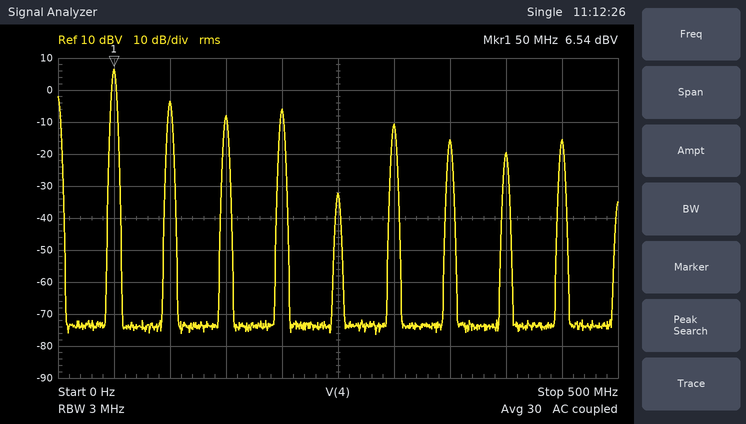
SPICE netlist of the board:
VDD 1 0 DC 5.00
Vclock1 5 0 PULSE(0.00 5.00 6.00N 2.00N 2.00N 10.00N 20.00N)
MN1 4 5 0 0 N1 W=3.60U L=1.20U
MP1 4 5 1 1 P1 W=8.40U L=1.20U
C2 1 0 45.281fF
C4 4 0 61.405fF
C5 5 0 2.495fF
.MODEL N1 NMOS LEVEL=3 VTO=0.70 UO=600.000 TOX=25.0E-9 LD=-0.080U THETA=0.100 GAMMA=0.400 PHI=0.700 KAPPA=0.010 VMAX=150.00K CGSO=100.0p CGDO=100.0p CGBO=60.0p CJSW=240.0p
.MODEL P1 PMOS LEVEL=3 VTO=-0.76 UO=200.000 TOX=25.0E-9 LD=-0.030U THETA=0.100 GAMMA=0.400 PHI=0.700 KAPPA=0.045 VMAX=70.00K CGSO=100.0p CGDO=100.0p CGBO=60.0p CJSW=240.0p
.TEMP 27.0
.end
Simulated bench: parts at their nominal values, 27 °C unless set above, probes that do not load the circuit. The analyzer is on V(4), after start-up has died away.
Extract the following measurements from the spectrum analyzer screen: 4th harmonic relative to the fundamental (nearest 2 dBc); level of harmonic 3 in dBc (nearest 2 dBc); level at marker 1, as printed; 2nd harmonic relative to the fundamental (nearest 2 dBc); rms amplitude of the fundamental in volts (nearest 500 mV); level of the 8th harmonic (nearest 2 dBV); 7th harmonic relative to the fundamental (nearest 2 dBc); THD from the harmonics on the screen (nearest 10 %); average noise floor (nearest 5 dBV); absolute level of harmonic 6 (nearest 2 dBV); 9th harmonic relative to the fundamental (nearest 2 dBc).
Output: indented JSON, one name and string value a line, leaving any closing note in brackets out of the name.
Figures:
{
  "4th harmonic relative to the fundamental": "-12 dBc",
  "level of harmonic 3 in dBc": "-14 dBc",
  "level at marker 1, as printed": "6.54 dBV",
  "2nd harmonic relative to the fundamental": "-10 dBc",
  "rms amplitude of the fundamental in volts": "2.0 V",
  "level of the 8th harmonic": "-20 dBV",
  "7th harmonic relative to the fundamental": "-22 dBc",
  "THD from the harmonics on the screen": "50 %",
  "average noise floor": "-75 dBV",
  "absolute level of harmonic 6": "-10 dBV",
  "9th harmonic relative to the fundamental": "-22 dBc"
}
